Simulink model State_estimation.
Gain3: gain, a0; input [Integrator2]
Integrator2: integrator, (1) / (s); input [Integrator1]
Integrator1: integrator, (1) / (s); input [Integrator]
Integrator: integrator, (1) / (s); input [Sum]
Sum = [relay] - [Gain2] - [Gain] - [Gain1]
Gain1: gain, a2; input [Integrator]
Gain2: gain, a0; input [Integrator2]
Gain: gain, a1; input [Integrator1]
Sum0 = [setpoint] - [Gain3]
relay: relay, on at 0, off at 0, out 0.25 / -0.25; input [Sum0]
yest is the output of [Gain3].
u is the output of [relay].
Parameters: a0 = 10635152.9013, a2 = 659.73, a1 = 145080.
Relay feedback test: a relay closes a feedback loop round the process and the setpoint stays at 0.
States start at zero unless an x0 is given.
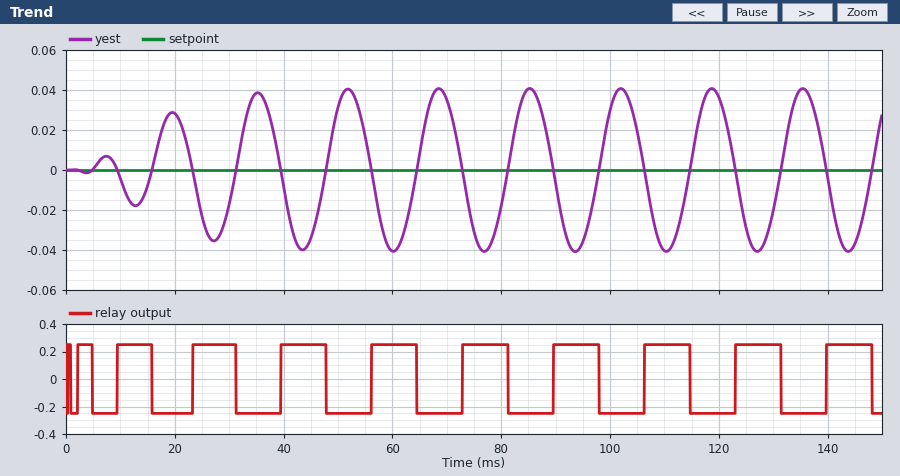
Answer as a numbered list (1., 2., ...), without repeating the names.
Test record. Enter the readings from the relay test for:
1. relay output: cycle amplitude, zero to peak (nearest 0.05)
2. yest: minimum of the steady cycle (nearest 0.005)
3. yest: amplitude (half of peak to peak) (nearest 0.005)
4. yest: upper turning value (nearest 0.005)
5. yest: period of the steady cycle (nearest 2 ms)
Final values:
1. 0.25
2. -0.040
3. 0.040
4. 0.040
5. 16 ms
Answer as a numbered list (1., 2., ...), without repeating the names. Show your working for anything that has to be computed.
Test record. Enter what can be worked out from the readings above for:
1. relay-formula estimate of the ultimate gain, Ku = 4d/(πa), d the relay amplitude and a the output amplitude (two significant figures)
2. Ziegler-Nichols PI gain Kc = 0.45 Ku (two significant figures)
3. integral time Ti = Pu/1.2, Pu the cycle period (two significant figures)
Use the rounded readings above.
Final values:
1. 4 × 0.25 / (π × 0.04) = 8.0
2. 0.45 × 8 = 3.6
3. 16 / 1.2 = 13 ms
